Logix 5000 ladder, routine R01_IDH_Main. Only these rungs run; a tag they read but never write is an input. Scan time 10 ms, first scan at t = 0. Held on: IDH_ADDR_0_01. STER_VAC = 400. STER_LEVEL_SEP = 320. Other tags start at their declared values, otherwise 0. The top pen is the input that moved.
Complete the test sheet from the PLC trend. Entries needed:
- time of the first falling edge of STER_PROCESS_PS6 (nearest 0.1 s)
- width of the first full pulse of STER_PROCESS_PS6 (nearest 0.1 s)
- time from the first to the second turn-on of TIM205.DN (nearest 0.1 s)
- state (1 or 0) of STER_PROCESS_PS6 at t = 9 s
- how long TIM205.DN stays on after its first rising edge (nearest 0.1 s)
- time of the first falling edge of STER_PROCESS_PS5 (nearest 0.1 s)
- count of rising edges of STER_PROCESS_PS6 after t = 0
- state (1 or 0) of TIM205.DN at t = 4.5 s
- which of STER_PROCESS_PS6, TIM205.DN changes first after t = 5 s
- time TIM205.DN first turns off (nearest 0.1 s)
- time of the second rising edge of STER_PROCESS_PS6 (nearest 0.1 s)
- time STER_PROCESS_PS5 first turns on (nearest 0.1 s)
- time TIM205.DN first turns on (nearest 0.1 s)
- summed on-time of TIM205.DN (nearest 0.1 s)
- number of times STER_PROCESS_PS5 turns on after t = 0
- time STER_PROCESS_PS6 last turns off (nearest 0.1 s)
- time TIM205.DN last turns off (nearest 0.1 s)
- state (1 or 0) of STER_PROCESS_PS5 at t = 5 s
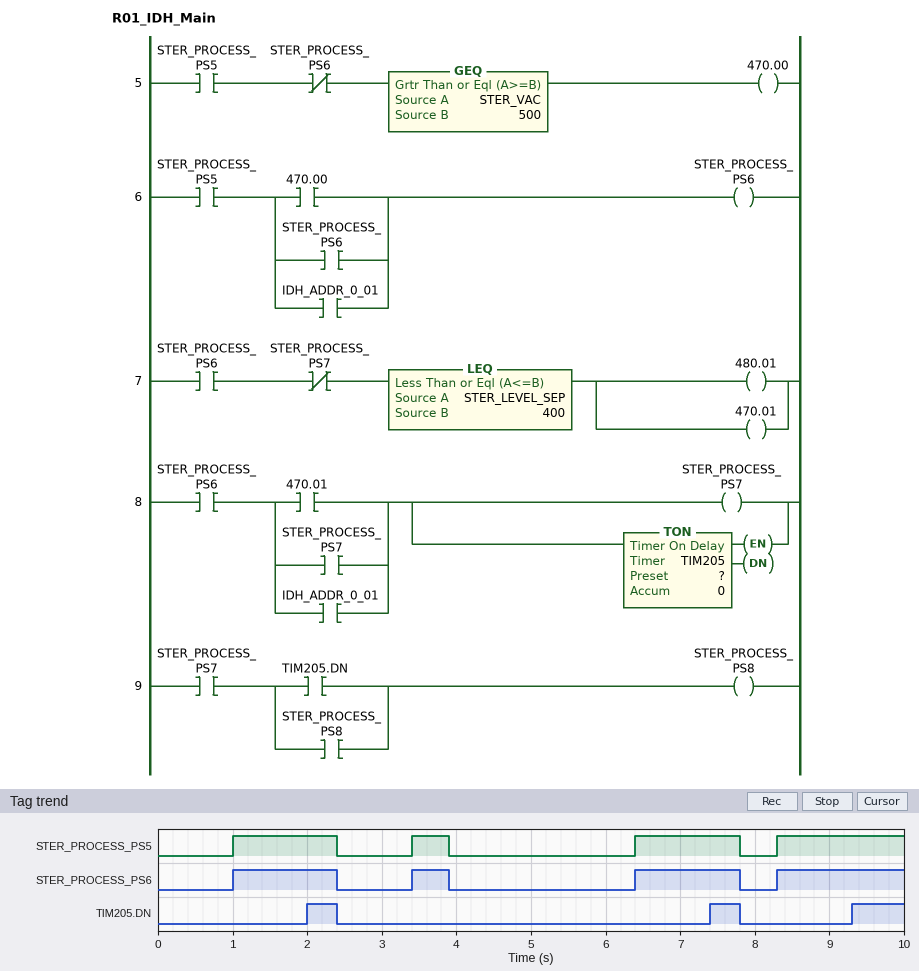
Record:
2.4 s
1.4 s
5.4 s
1
0.4 s
2.4 s
4
0
STER_PROCESS_PS6
2.4 s
3.4 s
1.0 s
2.0 s
1.5 s
4
7.8 s
7.8 s
0
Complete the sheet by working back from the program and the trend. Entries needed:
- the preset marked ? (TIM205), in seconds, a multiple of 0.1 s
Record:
1.0 s
